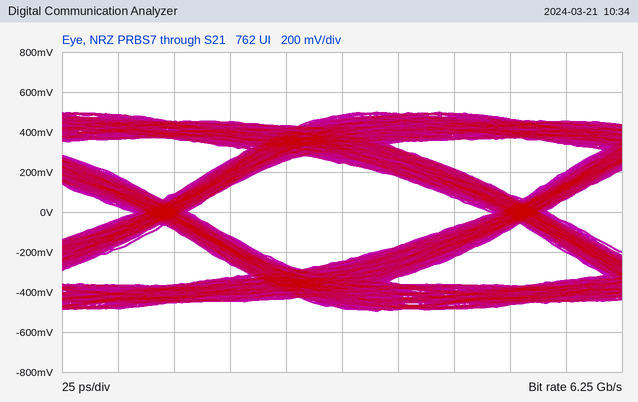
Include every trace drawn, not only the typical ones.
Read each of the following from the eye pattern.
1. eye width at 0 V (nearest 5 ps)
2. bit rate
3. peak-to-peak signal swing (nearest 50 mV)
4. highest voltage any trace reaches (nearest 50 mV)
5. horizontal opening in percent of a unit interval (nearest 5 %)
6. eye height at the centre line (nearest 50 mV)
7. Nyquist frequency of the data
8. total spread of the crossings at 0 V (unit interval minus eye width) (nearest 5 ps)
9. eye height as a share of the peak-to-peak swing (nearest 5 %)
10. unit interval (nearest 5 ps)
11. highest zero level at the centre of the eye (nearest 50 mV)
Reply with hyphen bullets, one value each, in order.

- 135 ps
- 6.25 Gb/s
- 1.00 V
- 500 mV
- 85 %
- 500 mV
- 3.125 GHz
- 25 ps
- 50 %
- 160 ps
- -250 mV
